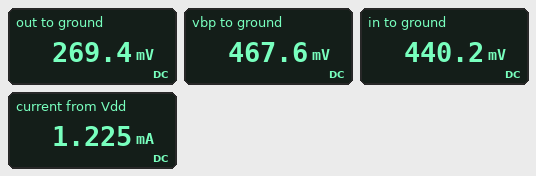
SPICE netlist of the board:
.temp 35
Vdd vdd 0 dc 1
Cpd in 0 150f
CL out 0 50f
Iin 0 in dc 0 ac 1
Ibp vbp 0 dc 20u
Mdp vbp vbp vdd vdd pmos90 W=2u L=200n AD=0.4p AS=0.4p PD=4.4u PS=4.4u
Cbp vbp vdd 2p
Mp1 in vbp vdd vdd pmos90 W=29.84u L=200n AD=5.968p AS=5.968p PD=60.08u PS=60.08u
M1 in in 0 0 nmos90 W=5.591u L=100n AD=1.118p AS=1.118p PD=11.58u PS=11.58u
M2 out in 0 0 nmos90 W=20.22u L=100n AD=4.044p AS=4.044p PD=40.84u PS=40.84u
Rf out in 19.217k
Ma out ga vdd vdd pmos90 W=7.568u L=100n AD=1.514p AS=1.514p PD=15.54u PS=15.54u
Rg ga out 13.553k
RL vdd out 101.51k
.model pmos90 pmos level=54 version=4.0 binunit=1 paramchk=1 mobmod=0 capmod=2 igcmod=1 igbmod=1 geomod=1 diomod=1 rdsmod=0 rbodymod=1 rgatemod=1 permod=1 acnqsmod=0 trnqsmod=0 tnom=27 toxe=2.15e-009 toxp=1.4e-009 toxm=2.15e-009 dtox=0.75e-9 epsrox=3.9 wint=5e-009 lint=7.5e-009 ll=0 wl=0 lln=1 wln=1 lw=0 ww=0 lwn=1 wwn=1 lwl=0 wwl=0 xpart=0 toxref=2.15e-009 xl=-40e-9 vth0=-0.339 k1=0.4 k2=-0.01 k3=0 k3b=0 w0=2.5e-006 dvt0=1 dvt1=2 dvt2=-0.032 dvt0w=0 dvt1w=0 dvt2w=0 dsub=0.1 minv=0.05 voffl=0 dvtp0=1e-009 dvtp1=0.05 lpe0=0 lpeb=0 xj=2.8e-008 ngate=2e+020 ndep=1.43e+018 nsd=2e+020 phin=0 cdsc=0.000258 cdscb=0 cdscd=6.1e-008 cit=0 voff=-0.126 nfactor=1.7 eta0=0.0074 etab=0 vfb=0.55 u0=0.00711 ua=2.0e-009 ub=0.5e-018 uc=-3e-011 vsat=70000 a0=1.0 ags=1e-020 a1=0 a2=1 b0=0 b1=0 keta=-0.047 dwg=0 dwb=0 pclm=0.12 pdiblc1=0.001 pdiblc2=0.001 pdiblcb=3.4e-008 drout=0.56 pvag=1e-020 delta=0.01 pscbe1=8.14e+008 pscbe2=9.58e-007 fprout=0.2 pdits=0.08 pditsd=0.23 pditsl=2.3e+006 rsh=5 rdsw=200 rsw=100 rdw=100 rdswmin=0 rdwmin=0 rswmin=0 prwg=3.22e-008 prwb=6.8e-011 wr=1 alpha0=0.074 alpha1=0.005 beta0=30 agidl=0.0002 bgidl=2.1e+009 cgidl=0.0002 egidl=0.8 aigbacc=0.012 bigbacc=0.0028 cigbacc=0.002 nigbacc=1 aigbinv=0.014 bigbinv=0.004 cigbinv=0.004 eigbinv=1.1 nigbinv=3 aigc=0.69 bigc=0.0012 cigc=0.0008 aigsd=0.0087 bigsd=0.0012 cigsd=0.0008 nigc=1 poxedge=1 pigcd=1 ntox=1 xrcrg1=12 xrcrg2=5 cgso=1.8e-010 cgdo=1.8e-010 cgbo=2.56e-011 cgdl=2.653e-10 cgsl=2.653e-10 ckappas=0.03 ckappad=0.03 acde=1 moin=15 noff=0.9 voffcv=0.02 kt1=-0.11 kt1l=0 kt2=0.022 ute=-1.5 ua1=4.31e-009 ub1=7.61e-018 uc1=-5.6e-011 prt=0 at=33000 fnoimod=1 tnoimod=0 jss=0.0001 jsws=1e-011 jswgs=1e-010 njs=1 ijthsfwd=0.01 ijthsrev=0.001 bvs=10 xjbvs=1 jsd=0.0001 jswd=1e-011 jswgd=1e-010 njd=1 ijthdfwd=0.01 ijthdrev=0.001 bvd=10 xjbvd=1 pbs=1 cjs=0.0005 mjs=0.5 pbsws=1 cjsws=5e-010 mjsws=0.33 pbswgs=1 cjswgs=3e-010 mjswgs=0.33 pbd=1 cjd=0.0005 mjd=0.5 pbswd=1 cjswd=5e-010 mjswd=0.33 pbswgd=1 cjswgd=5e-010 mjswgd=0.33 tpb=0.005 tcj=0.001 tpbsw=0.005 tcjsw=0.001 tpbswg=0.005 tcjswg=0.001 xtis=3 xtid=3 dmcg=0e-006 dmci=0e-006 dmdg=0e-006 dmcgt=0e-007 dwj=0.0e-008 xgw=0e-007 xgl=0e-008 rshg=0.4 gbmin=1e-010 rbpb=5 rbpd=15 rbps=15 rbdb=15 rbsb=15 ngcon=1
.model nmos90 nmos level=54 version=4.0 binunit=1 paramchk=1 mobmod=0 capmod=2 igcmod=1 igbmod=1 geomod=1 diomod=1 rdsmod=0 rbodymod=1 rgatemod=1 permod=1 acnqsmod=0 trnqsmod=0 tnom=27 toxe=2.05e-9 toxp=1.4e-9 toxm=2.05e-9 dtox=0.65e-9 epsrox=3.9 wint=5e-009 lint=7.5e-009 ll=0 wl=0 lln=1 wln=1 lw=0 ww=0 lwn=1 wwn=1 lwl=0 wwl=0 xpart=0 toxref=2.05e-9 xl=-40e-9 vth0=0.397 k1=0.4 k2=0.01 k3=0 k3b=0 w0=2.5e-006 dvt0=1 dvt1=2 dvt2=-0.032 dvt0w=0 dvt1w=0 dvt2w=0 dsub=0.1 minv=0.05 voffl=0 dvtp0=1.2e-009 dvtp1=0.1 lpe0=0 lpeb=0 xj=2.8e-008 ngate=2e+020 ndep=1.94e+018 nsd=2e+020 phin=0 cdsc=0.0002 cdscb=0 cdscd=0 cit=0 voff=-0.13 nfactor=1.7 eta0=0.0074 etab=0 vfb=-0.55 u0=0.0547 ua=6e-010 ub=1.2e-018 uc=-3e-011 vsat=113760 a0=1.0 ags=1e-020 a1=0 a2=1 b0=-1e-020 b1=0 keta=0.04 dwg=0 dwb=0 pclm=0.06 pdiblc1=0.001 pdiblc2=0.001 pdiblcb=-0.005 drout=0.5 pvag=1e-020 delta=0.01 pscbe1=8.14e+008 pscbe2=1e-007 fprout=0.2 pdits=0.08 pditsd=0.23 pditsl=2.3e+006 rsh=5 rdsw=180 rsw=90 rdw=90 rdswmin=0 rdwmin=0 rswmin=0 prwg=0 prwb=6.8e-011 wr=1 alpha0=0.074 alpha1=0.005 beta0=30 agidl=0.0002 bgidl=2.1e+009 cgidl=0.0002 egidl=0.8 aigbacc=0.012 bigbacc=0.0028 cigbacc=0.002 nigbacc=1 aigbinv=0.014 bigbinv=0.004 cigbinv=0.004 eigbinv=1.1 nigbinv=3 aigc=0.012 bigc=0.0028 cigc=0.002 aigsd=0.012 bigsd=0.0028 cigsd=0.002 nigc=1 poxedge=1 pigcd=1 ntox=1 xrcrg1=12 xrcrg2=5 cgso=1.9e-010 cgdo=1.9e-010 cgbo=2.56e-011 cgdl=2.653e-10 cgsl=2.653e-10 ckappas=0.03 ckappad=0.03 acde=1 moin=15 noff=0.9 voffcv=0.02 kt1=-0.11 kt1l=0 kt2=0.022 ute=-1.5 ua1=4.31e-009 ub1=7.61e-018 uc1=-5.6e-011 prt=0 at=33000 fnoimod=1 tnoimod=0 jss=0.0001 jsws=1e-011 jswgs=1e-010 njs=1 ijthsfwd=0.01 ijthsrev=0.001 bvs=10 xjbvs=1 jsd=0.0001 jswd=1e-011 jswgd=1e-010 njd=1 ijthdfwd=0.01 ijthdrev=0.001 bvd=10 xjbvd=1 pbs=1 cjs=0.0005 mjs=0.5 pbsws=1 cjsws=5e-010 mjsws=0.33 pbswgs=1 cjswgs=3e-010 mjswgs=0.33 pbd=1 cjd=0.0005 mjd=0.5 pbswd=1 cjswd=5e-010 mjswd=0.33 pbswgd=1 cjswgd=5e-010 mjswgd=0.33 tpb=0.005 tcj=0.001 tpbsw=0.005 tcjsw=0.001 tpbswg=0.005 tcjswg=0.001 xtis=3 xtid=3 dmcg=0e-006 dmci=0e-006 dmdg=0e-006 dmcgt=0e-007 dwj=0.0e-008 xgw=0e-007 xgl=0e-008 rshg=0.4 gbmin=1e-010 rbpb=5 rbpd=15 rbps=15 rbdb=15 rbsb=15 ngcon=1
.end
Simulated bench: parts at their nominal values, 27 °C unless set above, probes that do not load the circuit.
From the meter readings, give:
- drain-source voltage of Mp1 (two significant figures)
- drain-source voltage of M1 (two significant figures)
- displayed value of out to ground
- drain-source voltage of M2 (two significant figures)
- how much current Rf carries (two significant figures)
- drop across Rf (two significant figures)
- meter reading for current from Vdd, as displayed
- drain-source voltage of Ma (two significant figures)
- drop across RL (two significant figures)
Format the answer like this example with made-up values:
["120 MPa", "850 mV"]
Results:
["-560 mV", "440 mV", "269.4 mV", "270 mV", "8.9 µA", "170 mV", "1.225 mA", "-730 mV", "730 mV"]
